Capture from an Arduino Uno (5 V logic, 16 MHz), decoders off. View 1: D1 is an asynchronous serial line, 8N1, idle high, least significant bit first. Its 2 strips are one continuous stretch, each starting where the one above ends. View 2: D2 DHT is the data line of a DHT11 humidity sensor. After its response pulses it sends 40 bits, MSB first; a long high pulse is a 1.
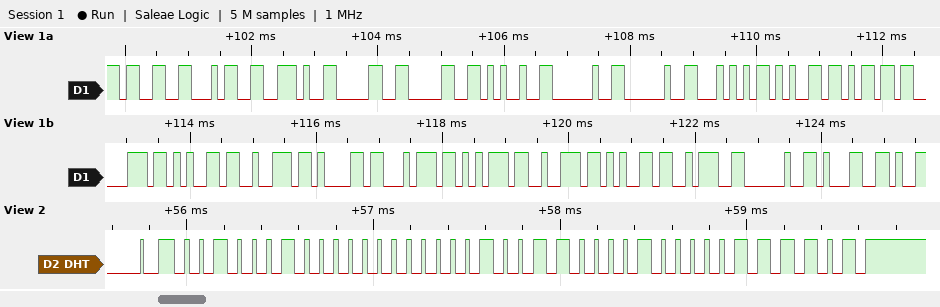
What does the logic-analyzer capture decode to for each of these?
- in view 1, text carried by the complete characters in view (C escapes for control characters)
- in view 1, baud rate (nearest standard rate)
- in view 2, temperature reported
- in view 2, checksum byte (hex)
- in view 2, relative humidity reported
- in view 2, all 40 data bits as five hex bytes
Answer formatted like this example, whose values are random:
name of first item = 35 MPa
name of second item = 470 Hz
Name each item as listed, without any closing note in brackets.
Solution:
in view 1, text carried by the complete characters in view = "34.00%  Temperature: 1"
in view 1, baud rate = 9600 baud
in view 2, temperature reported = 19.8 °C
in view 2, checksum byte = 0x3D
in view 2, relative humidity reported = 34 %
in view 2, all 40 data bits as five hex bytes = 22 00 13 08 3D
